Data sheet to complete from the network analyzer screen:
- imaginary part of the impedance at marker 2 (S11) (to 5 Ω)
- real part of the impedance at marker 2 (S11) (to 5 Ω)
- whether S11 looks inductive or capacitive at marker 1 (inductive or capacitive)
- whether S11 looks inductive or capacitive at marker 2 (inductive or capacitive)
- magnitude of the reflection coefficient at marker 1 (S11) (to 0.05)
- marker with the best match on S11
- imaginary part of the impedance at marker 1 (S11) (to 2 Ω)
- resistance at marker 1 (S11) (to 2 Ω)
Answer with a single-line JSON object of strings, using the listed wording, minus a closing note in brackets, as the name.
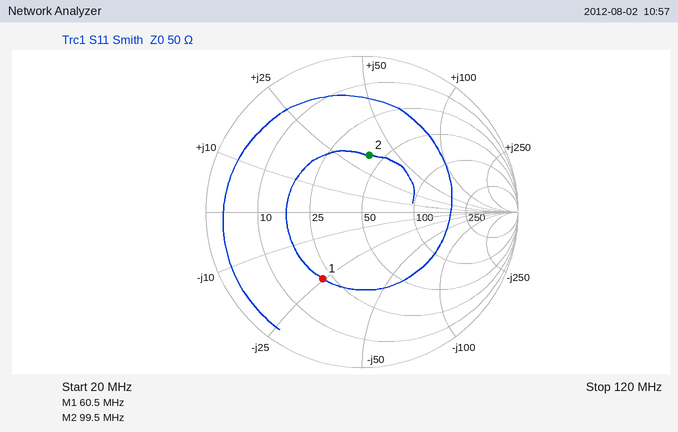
{"imaginary part of the impedance at marker 2 (S11)": "+35 Ω", "real part of the impedance at marker 2 (S11)": "40 Ω", "whether S11 looks inductive or capacitive at marker 1": "capacitive", "whether S11 looks inductive or capacitive at marker 2": "inductive", "magnitude of the reflection coefficient at marker 1 (S11)": "0.50", "marker with the best match on S11": "marker 2", "imaginary part of the impedance at marker 1 (S11)": "-24 Ω", "resistance at marker 1 (S11)": "22 Ω"}
